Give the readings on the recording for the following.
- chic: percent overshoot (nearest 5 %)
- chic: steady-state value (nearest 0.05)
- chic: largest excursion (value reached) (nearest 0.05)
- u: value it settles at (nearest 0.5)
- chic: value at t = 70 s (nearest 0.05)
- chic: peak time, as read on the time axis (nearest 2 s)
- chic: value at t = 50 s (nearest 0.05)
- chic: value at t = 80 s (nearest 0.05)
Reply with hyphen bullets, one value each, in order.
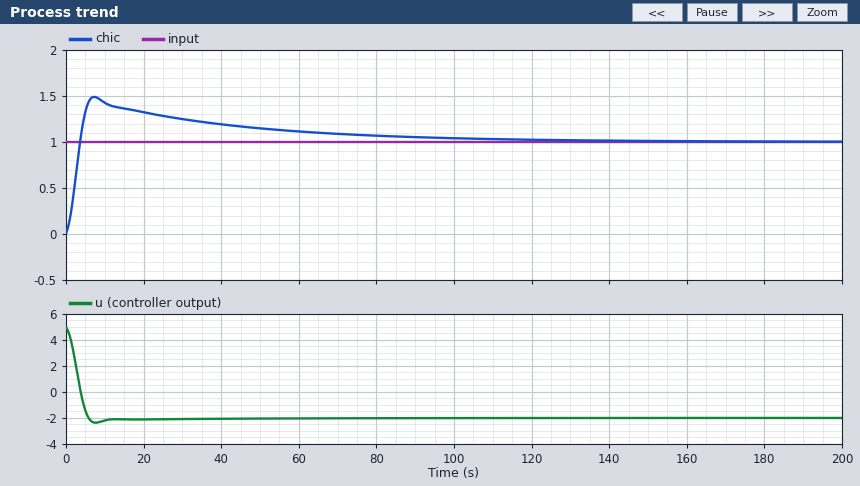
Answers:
- 50 %
- 1.00
- 1.50
- -2.0
- 1.10
- 8 s
- 1.15
- 1.05
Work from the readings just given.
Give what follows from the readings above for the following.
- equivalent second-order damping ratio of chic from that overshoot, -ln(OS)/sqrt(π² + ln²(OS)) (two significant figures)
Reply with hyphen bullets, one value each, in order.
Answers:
- 0.22
